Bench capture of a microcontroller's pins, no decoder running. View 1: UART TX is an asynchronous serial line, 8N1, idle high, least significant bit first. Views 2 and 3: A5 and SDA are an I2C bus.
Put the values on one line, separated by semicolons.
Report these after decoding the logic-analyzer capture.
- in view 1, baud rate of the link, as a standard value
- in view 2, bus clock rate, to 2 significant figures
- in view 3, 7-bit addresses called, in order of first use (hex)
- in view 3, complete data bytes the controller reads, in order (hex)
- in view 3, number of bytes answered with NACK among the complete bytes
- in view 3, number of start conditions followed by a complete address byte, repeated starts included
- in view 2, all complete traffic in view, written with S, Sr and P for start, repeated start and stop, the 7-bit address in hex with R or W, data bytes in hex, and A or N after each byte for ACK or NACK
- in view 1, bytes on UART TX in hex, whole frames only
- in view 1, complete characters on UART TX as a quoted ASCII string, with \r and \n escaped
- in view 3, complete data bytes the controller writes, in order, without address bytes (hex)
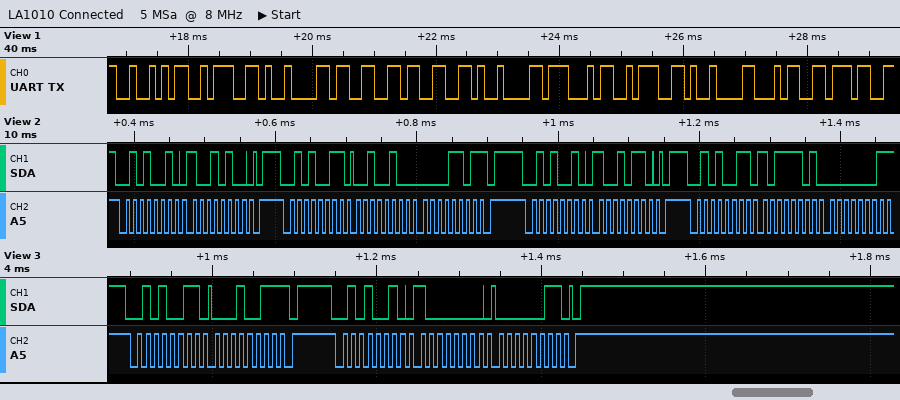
9600 baud; 100 kHz; 0x29; 13; 1; 2; S 29W A 94 A P S 29R A 24 A 0D N P S 29W A 96 A P S 29R A BD A 01 N; 52 3A 09 33 33 09 47 3A 09 34 37; "R:\t33\tG:\t47"; 80 03
